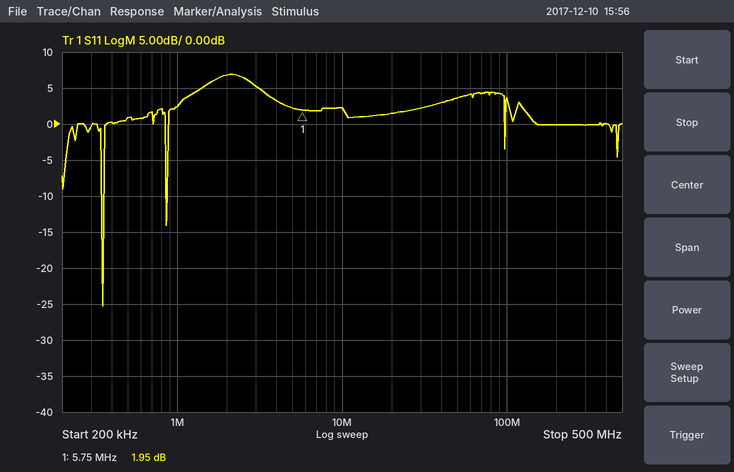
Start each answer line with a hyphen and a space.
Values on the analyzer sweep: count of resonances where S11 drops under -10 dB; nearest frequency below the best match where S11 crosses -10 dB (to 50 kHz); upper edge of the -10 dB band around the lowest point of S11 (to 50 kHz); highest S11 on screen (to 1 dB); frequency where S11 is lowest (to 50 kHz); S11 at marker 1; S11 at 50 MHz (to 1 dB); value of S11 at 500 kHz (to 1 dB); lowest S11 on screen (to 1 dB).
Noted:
- 2
- 350 kHz
- 350 kHz
- 7 dB
- 350 kHz
- 1.95 dB
- 4 dB
- 1 dB
- -25 dB
